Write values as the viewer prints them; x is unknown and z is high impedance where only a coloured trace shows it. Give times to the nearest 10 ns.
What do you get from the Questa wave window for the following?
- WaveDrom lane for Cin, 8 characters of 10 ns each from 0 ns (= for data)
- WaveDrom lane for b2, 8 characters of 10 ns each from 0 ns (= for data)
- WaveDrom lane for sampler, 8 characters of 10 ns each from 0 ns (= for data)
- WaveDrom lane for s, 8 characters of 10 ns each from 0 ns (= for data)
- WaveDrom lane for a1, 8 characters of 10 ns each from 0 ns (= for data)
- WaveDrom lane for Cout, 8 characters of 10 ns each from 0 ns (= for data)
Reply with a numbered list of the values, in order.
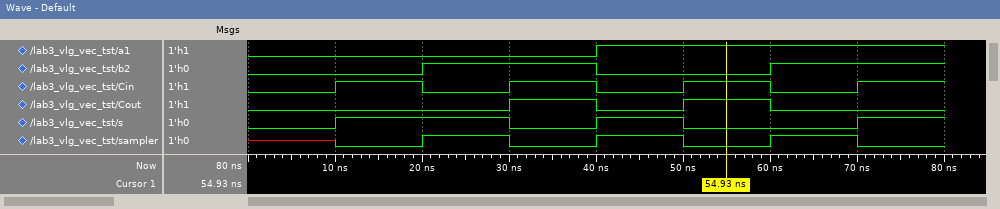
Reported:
1. {name: 'Cin', wave: '01010101'}
2. {name: 'b2', wave: '0.1.0.1.'}
3. {name: 'sampler', wave: 'x0101010'}
4. {name: 's', wave: '01.010.1'}
5. {name: 'a1', wave: '0...1...'}
6. {name: 'Cout', wave: '0..1010.'}
